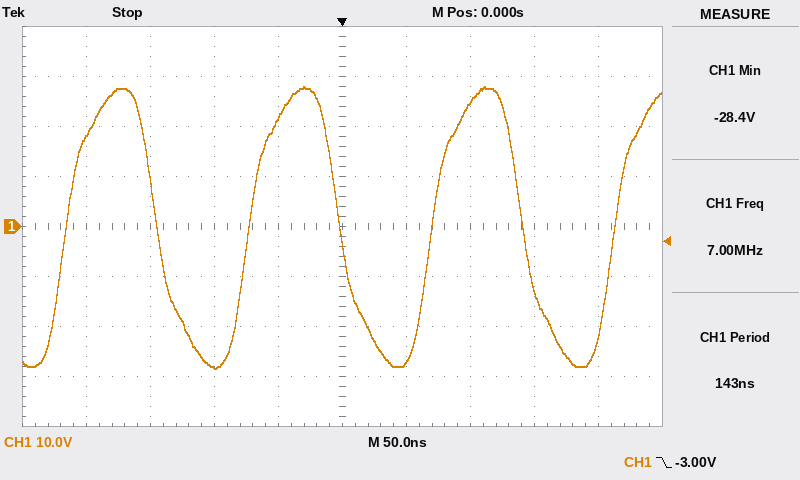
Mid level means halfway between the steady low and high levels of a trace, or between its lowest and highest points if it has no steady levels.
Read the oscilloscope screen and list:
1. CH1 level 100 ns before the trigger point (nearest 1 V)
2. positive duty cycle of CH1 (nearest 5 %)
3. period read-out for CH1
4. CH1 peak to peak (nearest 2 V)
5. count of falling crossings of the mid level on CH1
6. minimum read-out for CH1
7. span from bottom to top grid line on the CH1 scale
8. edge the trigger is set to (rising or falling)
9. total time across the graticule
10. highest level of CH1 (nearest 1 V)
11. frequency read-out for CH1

-28 V
50 %
143 ns
56 V
3
-28.4 V
80 V
falling
500 ns
28 V
7.00 MHz
